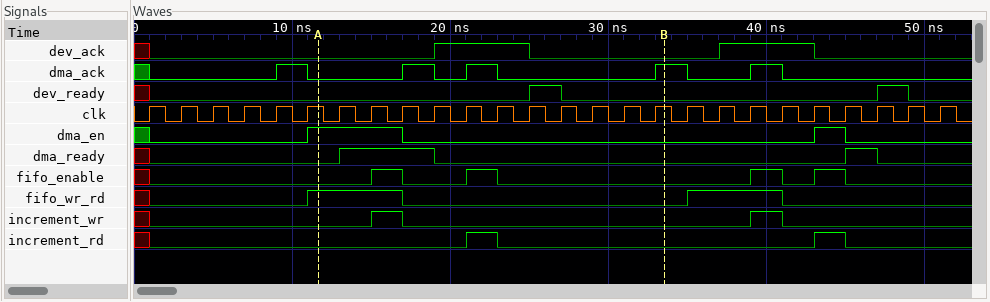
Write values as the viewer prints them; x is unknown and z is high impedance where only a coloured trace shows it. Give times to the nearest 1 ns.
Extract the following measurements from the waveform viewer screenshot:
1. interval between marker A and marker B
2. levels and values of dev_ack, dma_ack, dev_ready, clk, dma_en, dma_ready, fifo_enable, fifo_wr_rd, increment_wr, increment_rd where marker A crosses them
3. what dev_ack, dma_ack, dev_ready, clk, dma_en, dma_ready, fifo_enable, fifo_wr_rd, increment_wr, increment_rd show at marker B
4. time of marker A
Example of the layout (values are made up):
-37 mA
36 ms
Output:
22 ns
dev_ack=0, dma_ack=0, dev_ready=0, clk=1, dma_en=1, dma_ready=0, fifo_enable=0, fifo_wr_rd=1, increment_wr=0, increment_rd=0
dev_ack=0, dma_ack=1, dev_ready=0, clk=1, dma_en=0, dma_ready=0, fifo_enable=0, fifo_wr_rd=0, increment_wr=0, increment_rd=0
12 ns
